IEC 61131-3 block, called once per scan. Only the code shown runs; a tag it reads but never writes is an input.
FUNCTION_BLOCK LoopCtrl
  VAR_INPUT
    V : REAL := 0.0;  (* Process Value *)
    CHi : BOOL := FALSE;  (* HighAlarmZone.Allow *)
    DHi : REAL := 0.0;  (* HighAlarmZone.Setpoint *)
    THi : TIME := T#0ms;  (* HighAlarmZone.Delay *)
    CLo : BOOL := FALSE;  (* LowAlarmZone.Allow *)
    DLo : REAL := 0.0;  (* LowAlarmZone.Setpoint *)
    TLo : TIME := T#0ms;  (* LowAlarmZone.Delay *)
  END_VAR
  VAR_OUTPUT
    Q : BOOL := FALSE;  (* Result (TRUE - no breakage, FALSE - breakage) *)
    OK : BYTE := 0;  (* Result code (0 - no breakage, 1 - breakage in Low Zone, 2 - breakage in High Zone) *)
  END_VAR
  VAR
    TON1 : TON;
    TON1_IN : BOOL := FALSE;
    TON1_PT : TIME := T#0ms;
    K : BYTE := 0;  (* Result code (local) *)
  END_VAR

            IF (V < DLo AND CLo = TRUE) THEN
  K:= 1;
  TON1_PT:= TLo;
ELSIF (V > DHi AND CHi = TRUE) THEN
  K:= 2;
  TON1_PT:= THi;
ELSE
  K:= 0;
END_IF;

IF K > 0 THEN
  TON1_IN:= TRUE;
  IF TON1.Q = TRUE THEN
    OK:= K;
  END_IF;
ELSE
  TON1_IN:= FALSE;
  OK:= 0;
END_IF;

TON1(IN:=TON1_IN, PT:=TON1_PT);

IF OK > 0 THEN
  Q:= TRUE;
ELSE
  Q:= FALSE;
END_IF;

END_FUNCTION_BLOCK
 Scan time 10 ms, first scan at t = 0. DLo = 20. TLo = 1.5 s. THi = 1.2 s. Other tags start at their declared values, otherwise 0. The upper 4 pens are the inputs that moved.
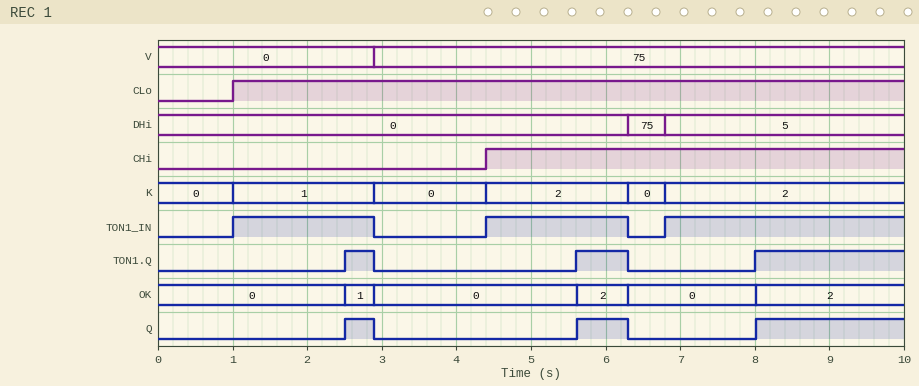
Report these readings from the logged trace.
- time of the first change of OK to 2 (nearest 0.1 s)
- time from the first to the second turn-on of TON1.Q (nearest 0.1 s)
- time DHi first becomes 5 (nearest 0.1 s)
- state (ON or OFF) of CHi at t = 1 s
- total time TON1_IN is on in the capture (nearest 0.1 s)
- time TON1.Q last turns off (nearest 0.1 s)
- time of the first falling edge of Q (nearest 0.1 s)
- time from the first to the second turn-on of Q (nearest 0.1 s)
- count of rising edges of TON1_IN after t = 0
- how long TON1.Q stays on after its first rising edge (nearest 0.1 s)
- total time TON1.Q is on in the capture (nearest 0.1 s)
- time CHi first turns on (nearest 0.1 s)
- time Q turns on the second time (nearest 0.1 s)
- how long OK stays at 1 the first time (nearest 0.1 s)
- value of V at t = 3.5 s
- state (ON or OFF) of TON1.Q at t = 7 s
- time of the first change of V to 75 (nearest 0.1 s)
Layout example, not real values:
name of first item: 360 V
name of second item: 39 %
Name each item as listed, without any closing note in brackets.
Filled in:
time of the first change of OK to 2: 5.6 s
time from the first to the second turn-on of TON1.Q: 3.1 s
time DHi first becomes 5: 6.8 s
state (ON or OFF) of CHi at t = 1 s: OFF
total time TON1_IN is on in the capture: 7.0 s
time TON1.Q last turns off: 6.3 s
time of the first falling edge of Q: 2.9 s
time from the first to the second turn-on of Q: 3.1 s
count of rising edges of TON1_IN after t = 0: 3
how long TON1.Q stays on after its first rising edge: 0.4 s
total time TON1.Q is on in the capture: 3.1 s
time CHi first turns on: 4.4 s
time Q turns on the second time: 5.6 s
how long OK stays at 1 the first time: 0.4 s
value of V at t = 3.5 s: 75
state (ON or OFF) of TON1.Q at t = 7 s: OFF
time of the first change of V to 75: 2.9 s
